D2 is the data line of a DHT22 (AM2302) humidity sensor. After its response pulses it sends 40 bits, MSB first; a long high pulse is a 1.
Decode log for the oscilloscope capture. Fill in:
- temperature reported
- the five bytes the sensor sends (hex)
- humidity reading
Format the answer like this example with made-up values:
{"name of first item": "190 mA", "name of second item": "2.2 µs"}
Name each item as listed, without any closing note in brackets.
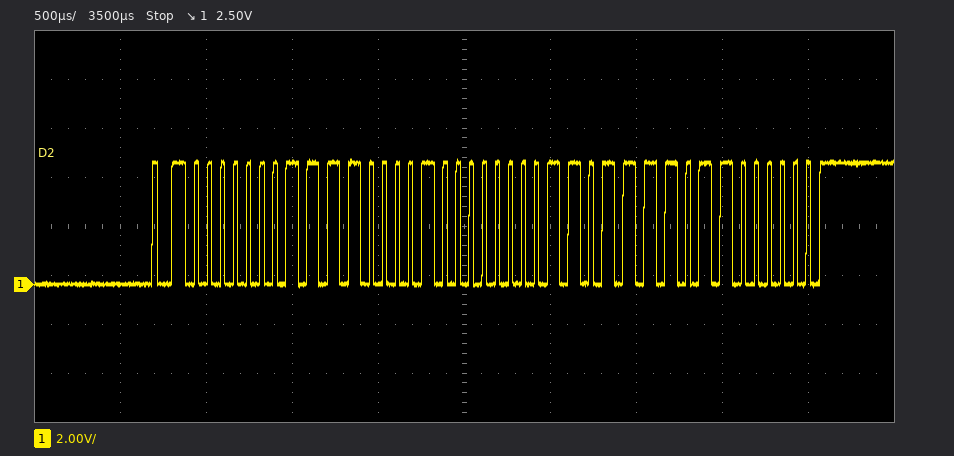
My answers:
{"temperature reported": "22.2 °C", "the five bytes the sensor sends": "01 E1 00 DE C0", "humidity reading": "48.1 %"}
